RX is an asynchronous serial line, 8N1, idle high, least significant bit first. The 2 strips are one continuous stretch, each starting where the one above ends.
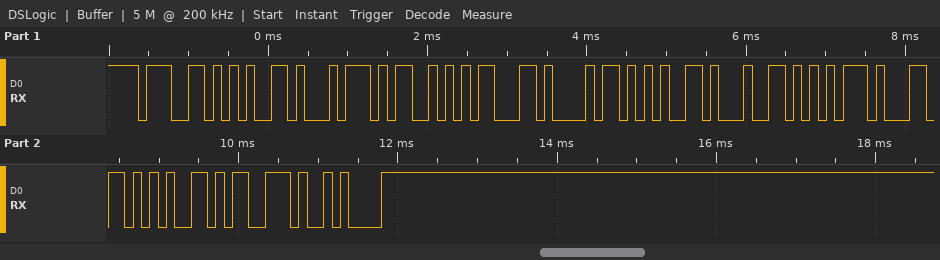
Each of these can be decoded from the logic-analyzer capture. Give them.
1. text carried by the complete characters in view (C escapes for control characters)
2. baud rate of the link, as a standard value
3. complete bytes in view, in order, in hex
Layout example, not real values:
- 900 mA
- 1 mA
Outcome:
- "getSchedules\n"
- 9600 baud
- 0x67 0x65 0x74 0x53 0x63 0x68 0x65 0x64 0x75 0x6C 0x65 0x73 0x0A
